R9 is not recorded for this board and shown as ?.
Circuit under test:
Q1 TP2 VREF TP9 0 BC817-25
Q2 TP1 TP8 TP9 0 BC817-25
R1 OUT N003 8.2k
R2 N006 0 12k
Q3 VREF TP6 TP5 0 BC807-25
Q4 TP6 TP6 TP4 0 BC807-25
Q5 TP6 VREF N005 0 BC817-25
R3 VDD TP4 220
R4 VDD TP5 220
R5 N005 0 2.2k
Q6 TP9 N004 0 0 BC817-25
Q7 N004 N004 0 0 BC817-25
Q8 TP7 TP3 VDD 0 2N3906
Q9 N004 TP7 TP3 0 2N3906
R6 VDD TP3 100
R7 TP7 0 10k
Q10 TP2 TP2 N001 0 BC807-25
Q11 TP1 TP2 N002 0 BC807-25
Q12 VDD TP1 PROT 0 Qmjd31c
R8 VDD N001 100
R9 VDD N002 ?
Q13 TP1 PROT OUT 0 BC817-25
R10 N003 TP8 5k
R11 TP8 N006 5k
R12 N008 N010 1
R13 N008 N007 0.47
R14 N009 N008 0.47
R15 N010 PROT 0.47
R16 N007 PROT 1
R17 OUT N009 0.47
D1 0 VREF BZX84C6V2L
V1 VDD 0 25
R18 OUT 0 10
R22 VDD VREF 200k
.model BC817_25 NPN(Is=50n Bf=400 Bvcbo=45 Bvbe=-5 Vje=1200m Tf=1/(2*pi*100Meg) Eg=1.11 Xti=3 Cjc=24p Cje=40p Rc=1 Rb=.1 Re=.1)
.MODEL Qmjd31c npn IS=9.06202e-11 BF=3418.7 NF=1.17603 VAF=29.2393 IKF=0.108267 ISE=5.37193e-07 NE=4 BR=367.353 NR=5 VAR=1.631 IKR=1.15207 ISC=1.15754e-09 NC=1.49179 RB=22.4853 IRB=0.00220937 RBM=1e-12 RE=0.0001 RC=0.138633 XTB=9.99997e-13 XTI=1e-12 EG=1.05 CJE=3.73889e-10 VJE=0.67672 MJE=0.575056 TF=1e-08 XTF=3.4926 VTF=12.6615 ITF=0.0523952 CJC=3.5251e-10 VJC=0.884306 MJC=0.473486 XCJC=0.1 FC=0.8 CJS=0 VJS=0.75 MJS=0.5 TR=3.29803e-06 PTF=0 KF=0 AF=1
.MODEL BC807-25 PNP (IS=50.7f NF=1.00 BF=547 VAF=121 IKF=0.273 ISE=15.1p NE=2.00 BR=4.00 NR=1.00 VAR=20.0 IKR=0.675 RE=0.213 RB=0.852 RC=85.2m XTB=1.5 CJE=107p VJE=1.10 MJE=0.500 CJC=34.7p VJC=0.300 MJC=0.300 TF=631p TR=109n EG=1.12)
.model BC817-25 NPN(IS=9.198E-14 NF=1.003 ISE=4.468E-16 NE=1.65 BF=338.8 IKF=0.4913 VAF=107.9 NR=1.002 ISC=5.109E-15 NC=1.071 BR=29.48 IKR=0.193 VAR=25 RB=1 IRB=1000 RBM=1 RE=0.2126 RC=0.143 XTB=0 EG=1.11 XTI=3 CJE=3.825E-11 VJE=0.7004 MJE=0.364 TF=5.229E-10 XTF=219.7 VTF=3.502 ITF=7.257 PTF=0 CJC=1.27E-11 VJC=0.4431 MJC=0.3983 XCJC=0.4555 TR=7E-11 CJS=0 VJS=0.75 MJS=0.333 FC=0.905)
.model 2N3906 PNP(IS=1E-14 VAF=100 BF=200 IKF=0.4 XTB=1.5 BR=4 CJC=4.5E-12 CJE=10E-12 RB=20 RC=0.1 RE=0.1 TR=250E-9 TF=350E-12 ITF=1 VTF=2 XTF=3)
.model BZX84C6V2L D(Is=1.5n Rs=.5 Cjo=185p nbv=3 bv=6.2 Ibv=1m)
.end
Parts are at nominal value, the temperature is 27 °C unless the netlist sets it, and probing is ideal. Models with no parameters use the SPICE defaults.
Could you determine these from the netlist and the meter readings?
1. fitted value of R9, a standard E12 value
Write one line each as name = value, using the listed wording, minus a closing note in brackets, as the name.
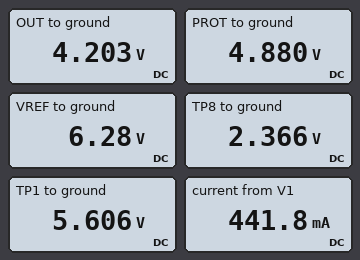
fitted value of R9, a standard E12 value = 39 Ω
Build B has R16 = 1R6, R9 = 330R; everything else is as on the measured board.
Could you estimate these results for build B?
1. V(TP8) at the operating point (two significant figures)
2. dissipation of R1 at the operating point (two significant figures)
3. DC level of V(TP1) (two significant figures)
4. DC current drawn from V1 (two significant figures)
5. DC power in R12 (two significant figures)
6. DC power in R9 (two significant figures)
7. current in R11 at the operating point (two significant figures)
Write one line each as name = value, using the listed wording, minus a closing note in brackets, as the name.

V(TP8) at the operating point = 1.9 V
dissipation of R1 at the operating point = 100 µW
DC level of V(TP1) = 4.7 V
DC current drawn from V1 = 360 mA
DC power in R12 = 39 mW
DC power in R9 = 1.6 mW
current in R11 at the operating point = 110 µA
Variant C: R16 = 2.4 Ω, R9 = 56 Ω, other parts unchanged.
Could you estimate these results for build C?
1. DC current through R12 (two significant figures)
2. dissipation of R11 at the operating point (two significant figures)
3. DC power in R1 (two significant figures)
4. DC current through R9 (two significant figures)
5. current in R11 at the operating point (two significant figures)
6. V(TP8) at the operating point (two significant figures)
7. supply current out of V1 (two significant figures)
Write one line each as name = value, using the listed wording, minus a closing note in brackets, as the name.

DC current through R12 = 230 mA
dissipation of R11 at the operating point = 71 µW
DC power in R1 = 120 µW
DC current through R9 = 12 mA
current in R11 at the operating point = 120 µA
V(TP8) at the operating point = 2.0 V
supply current out of V1 = 380 mA
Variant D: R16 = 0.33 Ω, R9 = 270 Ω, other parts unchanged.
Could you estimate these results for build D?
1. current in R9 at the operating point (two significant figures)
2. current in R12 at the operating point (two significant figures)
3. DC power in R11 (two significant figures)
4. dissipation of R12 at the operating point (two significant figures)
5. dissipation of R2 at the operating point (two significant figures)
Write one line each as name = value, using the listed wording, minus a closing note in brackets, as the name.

current in R9 at the operating point = 2.7 mA
current in R12 at the operating point = 150 mA
DC power in R11 = 98 µW
dissipation of R12 at the operating point = 22 mW
dissipation of R2 at the operating point = 240 µW
